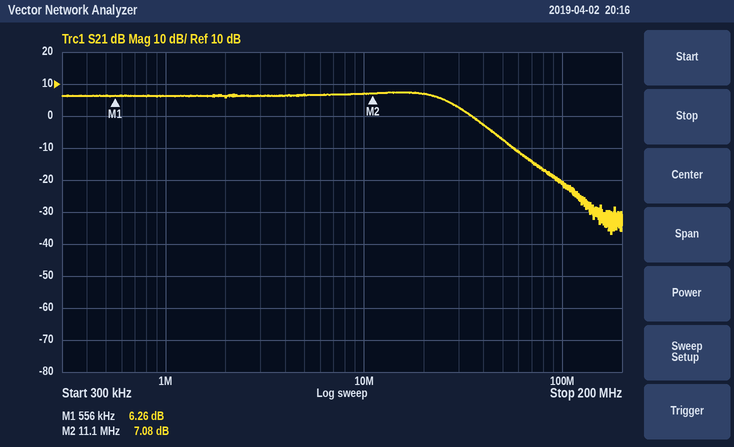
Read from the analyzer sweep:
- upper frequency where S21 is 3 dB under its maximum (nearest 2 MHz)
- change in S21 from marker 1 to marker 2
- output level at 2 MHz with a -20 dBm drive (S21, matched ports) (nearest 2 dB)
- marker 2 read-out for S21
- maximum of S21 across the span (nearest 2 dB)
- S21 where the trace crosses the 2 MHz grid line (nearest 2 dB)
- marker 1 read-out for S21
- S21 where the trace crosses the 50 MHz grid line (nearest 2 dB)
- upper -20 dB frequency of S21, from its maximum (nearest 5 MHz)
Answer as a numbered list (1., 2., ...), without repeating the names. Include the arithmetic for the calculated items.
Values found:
1. 26 MHz
2. 7.08 − (6.26) = 0.82 dB
3. -20 dBm + (6 dB) = -14 dBm
4. 7.08 dB
5. 8 dB
6. 6 dB
7. 6.26 dB
8. -8 dB
9. 65 MHz
